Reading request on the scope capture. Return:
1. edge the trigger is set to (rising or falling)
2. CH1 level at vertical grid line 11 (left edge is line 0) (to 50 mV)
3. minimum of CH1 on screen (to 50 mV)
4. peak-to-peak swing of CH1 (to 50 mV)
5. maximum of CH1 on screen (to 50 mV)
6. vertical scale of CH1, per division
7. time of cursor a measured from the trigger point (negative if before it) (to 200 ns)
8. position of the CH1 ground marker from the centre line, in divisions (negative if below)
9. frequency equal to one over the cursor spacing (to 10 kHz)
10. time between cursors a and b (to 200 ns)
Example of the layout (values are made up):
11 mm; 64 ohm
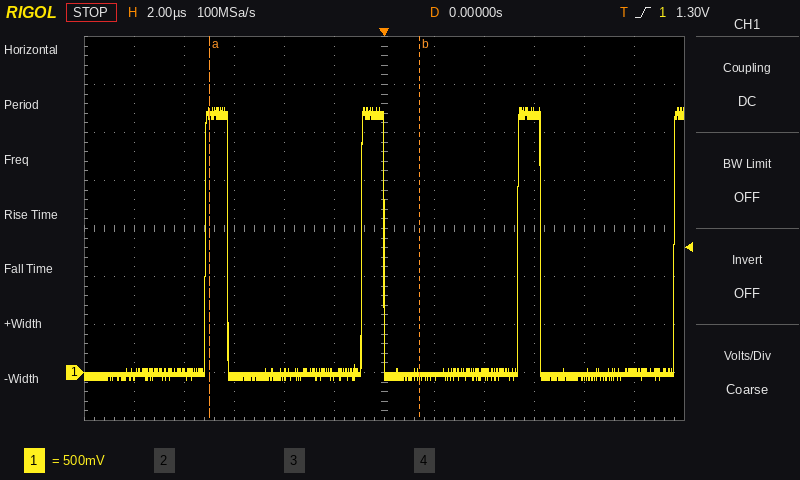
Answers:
rising; 0 mV; -100 mV; 2.85 V; 2.75 V; 500 mV; -7.0 µs; -3.0 div; 120 kHz; 8.4 µs
